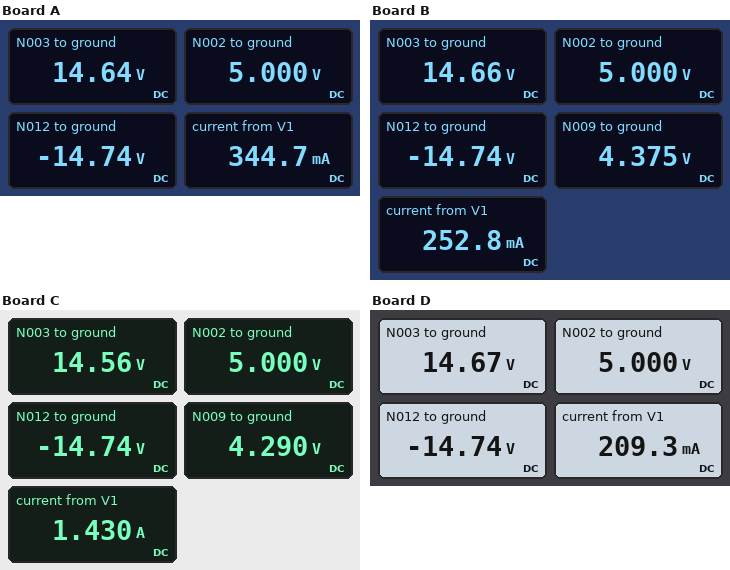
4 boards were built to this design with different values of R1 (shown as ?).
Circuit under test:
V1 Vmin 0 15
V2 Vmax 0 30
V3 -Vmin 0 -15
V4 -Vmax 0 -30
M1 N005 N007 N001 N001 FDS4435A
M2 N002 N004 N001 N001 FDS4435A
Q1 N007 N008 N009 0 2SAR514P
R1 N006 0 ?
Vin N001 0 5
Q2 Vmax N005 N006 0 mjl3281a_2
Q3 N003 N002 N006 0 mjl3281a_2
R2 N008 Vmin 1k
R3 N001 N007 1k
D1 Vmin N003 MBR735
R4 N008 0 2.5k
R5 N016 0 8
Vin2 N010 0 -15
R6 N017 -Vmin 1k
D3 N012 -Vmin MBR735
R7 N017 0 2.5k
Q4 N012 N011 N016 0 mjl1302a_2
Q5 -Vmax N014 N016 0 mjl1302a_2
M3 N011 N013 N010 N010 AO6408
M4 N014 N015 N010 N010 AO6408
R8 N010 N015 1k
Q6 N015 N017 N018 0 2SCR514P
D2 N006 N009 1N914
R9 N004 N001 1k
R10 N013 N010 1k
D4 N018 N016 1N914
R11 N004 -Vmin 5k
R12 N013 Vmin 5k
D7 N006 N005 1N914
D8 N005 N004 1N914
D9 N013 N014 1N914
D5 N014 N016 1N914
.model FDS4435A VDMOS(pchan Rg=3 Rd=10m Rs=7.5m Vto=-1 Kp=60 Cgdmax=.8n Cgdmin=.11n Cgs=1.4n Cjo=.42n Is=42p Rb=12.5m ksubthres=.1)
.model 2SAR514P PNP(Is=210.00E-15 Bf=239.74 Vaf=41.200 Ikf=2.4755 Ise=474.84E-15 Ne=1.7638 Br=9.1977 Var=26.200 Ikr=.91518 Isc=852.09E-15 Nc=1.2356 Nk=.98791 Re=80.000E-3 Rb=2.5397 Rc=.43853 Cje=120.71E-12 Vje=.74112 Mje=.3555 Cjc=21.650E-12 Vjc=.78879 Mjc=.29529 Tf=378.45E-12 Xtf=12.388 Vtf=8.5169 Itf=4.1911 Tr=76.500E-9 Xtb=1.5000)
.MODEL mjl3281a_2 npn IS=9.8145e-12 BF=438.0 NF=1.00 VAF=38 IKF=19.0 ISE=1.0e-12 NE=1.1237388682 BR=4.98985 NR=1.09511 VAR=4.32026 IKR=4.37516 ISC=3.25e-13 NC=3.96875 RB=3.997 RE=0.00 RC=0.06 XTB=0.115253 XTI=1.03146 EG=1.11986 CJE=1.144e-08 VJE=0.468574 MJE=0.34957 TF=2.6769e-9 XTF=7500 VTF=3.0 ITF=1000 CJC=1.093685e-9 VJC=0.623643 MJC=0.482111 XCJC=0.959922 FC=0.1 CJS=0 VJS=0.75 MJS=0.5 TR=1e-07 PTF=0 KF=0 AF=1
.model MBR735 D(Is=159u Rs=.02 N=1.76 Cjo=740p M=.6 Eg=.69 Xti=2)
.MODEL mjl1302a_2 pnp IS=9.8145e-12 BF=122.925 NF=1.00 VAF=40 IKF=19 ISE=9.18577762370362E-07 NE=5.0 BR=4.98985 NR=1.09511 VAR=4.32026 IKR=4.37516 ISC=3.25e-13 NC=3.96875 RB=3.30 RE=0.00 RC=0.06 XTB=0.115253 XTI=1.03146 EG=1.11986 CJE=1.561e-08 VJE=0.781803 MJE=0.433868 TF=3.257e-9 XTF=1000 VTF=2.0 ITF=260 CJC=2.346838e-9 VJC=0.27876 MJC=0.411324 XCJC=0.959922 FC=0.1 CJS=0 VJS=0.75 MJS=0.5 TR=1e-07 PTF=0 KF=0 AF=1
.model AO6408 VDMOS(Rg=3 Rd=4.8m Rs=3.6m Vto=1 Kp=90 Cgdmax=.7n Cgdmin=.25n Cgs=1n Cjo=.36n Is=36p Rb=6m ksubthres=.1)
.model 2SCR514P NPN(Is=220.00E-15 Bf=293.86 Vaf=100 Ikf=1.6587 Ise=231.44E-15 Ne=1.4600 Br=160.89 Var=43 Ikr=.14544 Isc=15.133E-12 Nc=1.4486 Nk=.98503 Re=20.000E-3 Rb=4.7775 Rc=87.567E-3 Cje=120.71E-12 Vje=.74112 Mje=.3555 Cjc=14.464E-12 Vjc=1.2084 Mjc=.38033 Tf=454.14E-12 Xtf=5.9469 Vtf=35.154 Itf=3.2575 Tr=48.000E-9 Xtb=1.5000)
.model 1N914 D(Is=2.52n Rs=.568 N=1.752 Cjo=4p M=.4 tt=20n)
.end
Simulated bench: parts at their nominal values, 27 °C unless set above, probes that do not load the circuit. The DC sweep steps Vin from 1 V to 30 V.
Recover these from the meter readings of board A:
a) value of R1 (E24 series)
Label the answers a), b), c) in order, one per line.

a) 13 Ω
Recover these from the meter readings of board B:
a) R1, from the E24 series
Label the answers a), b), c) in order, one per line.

a) 18 Ω
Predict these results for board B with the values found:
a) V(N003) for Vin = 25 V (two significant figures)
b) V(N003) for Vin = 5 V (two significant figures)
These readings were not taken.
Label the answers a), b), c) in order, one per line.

a) 24 V
b) 15 V
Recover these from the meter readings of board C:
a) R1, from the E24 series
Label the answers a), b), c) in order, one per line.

a) 3 Ω
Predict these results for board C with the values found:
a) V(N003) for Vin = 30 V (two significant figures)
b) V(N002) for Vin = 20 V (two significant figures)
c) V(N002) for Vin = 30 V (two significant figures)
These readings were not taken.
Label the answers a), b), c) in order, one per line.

a) 29 V
b) 20 V
c) 29 V
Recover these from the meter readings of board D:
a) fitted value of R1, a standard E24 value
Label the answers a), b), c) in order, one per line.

a) 22 Ω
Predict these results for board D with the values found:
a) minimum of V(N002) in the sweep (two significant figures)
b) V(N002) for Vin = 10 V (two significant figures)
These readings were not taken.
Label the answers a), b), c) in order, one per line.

a) 1.0 V
b) 10 V
